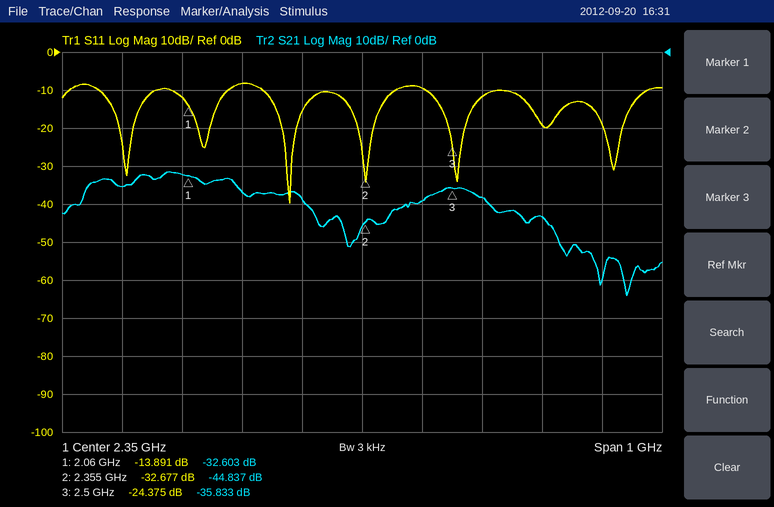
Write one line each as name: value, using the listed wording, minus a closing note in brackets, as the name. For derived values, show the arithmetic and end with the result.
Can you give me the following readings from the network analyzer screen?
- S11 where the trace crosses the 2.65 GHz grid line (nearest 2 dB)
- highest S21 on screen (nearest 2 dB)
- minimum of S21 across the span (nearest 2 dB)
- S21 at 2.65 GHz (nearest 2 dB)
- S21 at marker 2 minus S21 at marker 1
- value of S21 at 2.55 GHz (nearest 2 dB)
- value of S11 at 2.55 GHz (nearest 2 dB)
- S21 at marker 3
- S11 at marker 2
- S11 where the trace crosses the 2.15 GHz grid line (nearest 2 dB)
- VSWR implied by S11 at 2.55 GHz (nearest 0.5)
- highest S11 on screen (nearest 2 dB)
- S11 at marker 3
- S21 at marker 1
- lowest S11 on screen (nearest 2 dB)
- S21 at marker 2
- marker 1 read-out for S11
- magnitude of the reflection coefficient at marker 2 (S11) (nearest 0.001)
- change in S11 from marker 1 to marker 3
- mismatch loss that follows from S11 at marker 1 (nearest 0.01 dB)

S11 where the trace crosses the 2.65 GHz grid line: -20 dB
highest S21 on screen: -32 dB
minimum of S21 across the span: -64 dB
S21 at 2.65 GHz: -44 dB
S21 at marker 2 minus S21 at marker 1: -44.837 − (-32.603) = -12.234 dB
value of S21 at 2.55 GHz: -38 dB
value of S11 at 2.55 GHz: -12 dB
S21 at marker 3: -35.833 dB
S11 at marker 2: -32.677 dB
S11 where the trace crosses the 2.15 GHz grid line: -8 dB
VSWR implied by S11 at 2.55 GHz: |Γ| = 10^(-12/20) = 0.2512; VSWR = (1 + 0.2512)/(1 − 0.2512) ≈ 1.67, so 1.5 to the nearest 0.5
highest S11 on screen: -8 dB
S11 at marker 3: -24.375 dB
S21 at marker 1: -32.603 dB
lowest S11 on screen: -40 dB
S21 at marker 2: -44.837 dB
marker 1 read-out for S11: -13.891 dB
magnitude of the reflection coefficient at marker 2 (S11): 10^(-32.677/20) ≈ 0.023
change in S11 from marker 1 to marker 3: -24.375 − (-13.891) = -10.484 dB
mismatch loss that follows from S11 at marker 1: −10 log10(1 − 10^(-13.891/10)) ≈ 0.18 dB
